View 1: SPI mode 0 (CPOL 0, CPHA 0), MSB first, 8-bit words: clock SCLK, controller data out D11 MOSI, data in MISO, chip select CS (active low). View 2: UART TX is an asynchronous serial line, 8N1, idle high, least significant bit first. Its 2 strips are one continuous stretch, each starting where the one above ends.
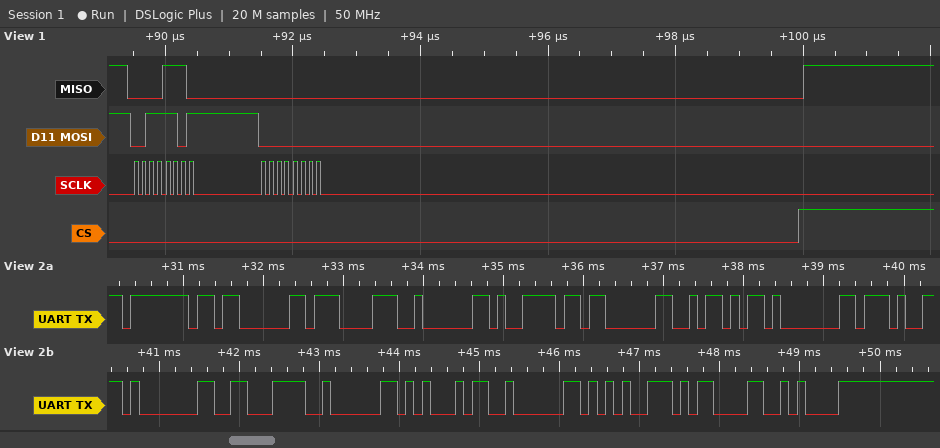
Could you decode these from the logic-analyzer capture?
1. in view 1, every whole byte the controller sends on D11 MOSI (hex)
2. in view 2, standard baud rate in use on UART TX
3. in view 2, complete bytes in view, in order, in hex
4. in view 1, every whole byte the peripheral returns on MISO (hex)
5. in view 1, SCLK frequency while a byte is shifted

3D 00
9600 baud
0x7F 0x03 0x87 0x02 0x79 0x03 0x5A 0x01 0x97 0x01 0xC6 0x02 0x45 0x02 0x95 0x0D 0x0A
0E 00
8 MHz
